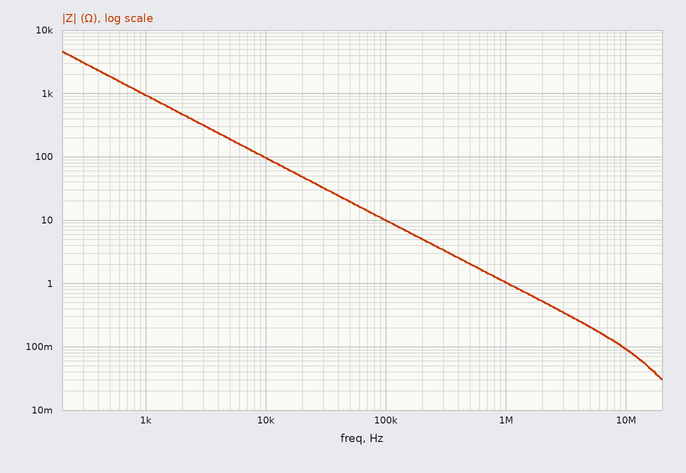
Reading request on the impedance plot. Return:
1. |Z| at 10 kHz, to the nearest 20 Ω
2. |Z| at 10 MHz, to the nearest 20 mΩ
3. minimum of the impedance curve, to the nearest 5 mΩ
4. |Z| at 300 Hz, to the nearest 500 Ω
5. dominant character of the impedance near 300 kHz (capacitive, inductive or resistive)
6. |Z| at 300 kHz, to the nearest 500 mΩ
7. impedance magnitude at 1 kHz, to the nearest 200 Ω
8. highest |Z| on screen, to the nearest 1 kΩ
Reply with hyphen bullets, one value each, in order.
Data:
- 100 Ω
- 100 mΩ
- 30 mΩ
- 3.0 kΩ
- capacitive
- 3.5 Ω
- 1.0 kΩ
- 5 kΩ
